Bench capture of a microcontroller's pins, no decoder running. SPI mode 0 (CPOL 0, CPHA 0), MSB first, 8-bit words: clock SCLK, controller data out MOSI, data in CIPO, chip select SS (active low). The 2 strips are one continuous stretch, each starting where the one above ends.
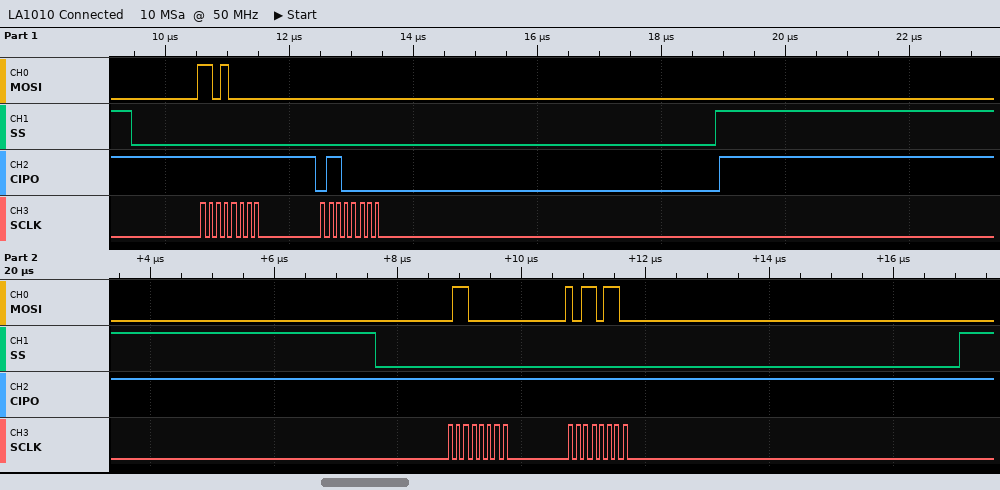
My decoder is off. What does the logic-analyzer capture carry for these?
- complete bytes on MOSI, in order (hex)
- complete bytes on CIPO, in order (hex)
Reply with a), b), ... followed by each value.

a) D0 00 60 B6
b) FF 60 FF FF
